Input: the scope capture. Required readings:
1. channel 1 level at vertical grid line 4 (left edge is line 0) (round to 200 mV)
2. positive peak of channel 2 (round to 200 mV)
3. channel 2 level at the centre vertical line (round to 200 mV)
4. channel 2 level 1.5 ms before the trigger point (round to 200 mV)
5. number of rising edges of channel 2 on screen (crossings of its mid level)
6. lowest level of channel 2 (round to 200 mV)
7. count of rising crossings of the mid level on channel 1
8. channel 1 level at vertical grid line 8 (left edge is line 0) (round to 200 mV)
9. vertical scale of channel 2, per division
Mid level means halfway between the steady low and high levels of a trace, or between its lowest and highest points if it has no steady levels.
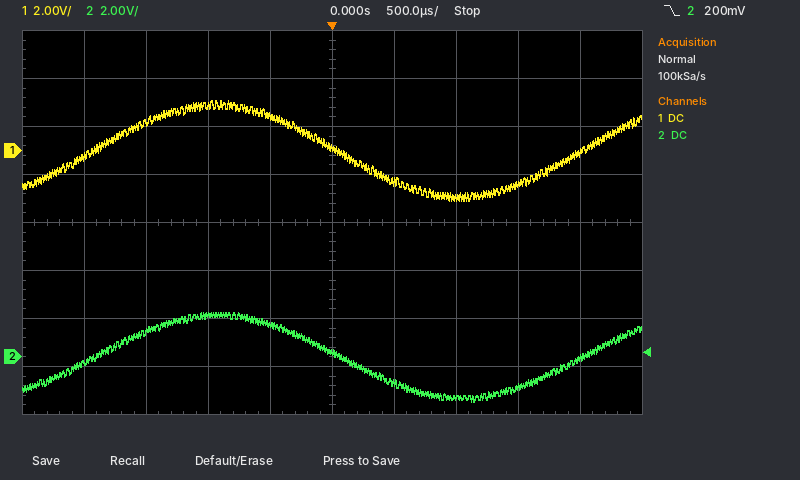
1.4 V
1.8 V
200 mV
1.0 V
2
-1.8 V
2
-1.4 V
2 V
